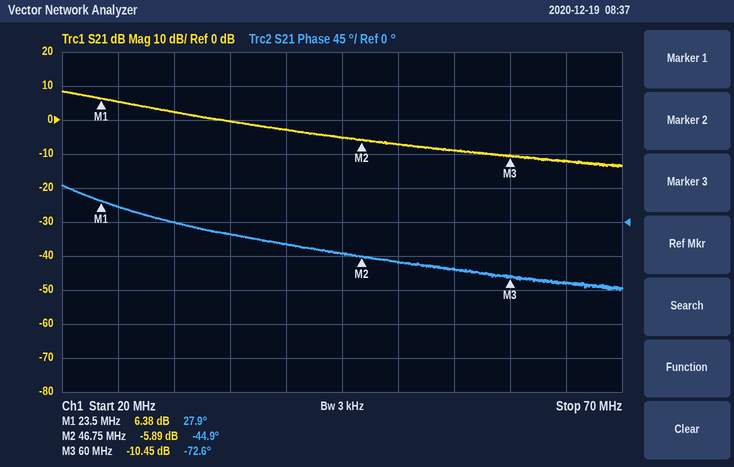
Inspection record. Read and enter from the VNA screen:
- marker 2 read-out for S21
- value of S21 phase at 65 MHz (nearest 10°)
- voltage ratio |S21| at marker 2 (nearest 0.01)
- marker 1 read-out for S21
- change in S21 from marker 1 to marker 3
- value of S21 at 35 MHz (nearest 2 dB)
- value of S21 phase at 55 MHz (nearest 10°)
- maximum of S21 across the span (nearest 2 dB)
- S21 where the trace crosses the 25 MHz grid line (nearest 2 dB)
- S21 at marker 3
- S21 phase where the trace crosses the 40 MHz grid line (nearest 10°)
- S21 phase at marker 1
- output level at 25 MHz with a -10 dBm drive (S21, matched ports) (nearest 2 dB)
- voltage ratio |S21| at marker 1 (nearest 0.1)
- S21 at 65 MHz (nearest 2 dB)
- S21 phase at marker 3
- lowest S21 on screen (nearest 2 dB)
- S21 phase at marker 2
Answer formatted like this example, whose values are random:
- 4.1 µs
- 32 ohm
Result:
- -5.89 dB
- -80°
- 0.51
- 6.38 dB
- -16.83 dB
- 0 dB
- -60°
- 8 dB
- 6 dB
- -10.45 dB
- -30°
- 27.9°
- -4 dBm
- 2.1
- -12 dB
- -72.6°
- -14 dB
- -44.9°
